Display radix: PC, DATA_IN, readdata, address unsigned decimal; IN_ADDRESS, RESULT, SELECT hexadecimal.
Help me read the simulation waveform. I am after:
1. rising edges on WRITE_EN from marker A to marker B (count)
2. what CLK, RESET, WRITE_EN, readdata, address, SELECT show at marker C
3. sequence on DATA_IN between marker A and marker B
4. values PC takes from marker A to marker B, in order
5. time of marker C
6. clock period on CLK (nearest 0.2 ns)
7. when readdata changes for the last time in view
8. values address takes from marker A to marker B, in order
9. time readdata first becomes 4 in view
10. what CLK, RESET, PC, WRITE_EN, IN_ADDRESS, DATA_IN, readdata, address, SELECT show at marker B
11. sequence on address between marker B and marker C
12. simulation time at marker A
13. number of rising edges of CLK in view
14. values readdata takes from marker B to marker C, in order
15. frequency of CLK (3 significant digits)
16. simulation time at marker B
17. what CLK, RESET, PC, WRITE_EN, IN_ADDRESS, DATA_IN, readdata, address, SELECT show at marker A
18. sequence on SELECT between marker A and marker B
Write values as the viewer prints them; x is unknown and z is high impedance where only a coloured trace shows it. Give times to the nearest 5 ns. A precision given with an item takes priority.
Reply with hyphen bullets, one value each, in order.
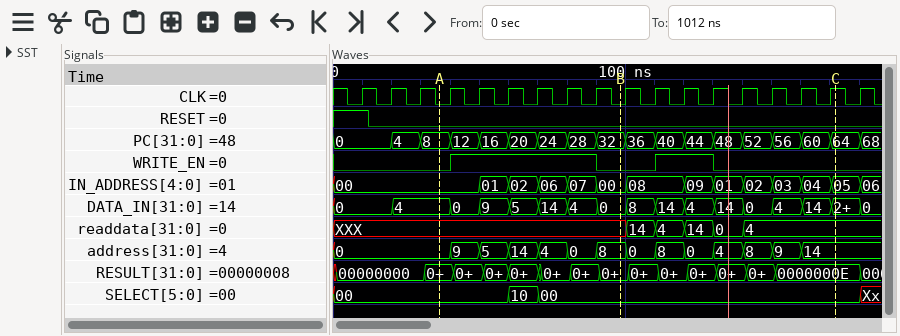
- 1
- CLK=1, RESET=0, WRITE_EN=0, readdata=4, address=14, SELECT=00
- 4, 0, 9, 5, 14, 4, 0
- 8, 12, 16, 20, 24, 28, 32
- 170 ns
- 10 ns
- 140 ns
- 0, 9, 5, 14, 4, 0, 8
- 110 ns
- CLK=0, RESET=0, PC=32, WRITE_EN=0, IN_ADDRESS=00, DATA_IN=0, readdata=XXX, address=8, SELECT=00
- 8, 0, 8, 0, 4, 8, 9, 14
- 35 ns
- 18
- XXX, 14, 4, 14, 0, 4
- 100 MHz
- 100 ns
- CLK=0, RESET=0, PC=8, WRITE_EN=0, IN_ADDRESS=00, DATA_IN=4, readdata=XXX, address=0, SELECT=00
- 00, 10, 00
